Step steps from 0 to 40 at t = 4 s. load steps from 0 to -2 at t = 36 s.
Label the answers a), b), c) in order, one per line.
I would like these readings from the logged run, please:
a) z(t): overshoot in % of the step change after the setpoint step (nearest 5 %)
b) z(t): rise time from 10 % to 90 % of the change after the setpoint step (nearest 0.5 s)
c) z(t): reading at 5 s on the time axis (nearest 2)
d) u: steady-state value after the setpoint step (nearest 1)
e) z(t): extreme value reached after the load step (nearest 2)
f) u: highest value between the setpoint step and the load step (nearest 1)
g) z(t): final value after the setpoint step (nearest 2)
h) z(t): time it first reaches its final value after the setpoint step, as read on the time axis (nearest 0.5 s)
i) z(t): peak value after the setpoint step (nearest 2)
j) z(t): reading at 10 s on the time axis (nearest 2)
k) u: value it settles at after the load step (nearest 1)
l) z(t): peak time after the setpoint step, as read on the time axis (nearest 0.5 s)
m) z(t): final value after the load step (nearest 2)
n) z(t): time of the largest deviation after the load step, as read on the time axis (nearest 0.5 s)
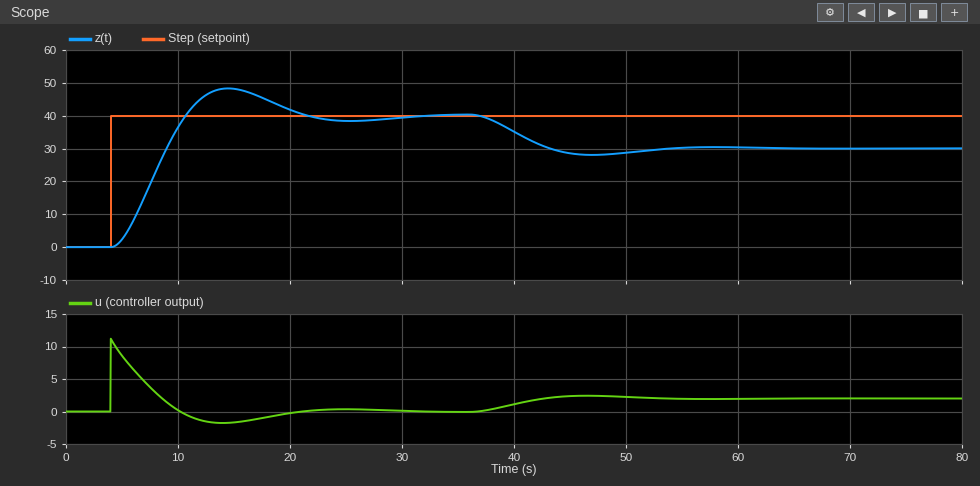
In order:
a) 20 %
b) 4.5 s
c) 2
d) 0
e) 28
f) 11
g) 40
h) 10.5 s
i) 48
j) 36
k) 2
l) 14.5 s
m) 30
n) 47.0 s
